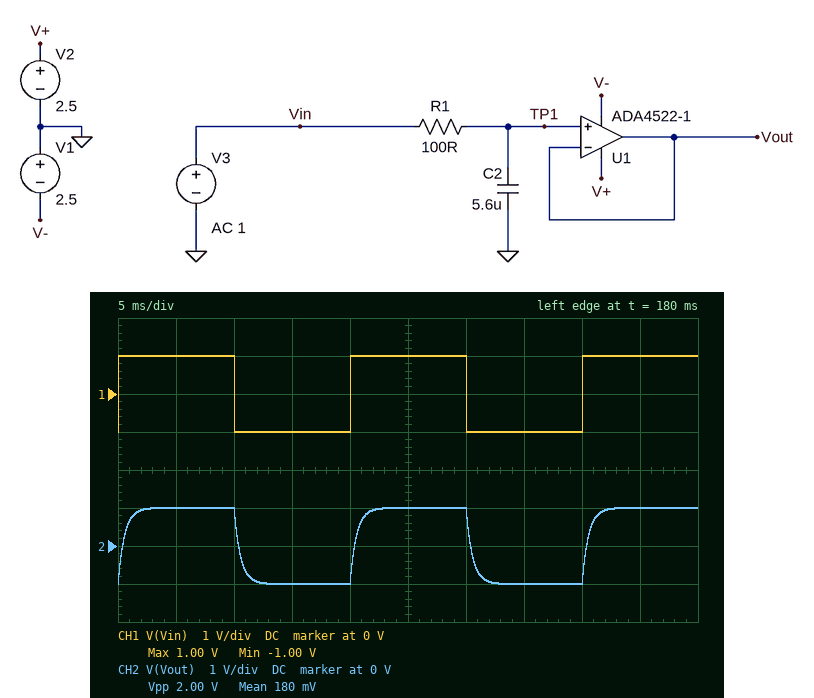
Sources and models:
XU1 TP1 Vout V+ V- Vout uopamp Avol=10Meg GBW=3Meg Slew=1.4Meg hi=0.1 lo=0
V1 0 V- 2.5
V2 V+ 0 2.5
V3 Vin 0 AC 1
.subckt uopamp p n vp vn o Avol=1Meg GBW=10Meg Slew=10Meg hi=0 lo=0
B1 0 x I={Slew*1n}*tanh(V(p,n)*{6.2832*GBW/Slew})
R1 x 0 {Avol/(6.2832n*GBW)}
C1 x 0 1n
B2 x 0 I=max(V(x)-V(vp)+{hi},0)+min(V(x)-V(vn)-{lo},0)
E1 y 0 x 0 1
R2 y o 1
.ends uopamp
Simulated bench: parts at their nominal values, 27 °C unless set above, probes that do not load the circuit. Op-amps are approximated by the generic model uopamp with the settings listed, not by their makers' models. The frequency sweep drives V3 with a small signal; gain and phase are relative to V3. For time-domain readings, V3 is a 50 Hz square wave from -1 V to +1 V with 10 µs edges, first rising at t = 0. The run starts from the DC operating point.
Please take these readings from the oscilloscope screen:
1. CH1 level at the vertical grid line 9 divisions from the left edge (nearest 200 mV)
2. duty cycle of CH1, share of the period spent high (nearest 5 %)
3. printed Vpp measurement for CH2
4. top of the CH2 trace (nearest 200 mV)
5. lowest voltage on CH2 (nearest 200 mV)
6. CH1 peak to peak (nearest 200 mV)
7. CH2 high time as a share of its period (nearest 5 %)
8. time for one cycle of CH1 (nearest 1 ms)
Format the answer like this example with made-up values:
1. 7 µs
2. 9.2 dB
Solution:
1. 1.0 V
2. 50 %
3. 2.00 V
4. 1.0 V
5. -1.0 V
6. 2.0 V
7. 50 %
8. 20 ms
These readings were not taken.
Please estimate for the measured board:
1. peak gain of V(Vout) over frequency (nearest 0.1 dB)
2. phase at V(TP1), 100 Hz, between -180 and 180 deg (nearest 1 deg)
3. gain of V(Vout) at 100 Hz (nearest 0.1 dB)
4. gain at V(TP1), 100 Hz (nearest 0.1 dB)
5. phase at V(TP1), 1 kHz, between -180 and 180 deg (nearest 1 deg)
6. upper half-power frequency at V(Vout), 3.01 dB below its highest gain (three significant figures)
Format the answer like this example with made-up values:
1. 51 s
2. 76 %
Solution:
1. 0 dB
2. -19 deg
3. -0.5 dB
4. -0.5 dB
5. -74 deg
6. 284 Hz
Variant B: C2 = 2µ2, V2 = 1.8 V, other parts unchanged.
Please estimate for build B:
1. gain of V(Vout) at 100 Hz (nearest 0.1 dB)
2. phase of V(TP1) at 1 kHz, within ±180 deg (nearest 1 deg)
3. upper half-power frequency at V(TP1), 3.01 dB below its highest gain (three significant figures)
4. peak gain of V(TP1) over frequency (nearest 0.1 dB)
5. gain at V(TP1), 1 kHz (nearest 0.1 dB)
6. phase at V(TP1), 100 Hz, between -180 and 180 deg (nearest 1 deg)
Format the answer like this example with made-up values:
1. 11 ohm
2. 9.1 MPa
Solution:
1. -0.1 dB
2. -54 deg
3. 723 Hz
4. 0 dB
5. -4.6 dB
6. -8 deg
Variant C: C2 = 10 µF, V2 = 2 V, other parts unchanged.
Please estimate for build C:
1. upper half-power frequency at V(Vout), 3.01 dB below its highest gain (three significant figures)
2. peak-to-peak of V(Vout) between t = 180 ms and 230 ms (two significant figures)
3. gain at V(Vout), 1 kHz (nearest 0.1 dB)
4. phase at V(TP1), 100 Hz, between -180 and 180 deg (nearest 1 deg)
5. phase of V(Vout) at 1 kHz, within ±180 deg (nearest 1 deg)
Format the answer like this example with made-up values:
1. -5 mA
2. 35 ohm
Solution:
1. 159 Hz
2. 2.0 V
3. -16.1 dB
4. -32 deg
5. -81 deg
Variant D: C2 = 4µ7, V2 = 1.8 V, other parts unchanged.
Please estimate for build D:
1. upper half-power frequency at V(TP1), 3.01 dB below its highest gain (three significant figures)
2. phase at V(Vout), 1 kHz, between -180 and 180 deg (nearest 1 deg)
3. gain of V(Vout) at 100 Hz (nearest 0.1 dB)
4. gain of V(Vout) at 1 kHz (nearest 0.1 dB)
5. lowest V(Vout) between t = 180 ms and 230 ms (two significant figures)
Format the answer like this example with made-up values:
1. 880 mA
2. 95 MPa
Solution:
1. 339 Hz
2. -71 deg
3. -0.4 dB
4. -9.9 dB
5. -1.0 V
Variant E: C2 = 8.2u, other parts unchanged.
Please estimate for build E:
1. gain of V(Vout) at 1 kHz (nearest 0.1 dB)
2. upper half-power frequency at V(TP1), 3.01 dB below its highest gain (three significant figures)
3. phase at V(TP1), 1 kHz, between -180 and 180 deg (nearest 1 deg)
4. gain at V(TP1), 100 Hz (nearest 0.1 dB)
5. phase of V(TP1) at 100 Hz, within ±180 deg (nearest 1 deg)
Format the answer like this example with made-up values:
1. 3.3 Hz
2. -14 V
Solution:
1. -14.4 dB
2. 194 Hz
3. -79 deg
4. -1.0 dB
5. -27 deg
